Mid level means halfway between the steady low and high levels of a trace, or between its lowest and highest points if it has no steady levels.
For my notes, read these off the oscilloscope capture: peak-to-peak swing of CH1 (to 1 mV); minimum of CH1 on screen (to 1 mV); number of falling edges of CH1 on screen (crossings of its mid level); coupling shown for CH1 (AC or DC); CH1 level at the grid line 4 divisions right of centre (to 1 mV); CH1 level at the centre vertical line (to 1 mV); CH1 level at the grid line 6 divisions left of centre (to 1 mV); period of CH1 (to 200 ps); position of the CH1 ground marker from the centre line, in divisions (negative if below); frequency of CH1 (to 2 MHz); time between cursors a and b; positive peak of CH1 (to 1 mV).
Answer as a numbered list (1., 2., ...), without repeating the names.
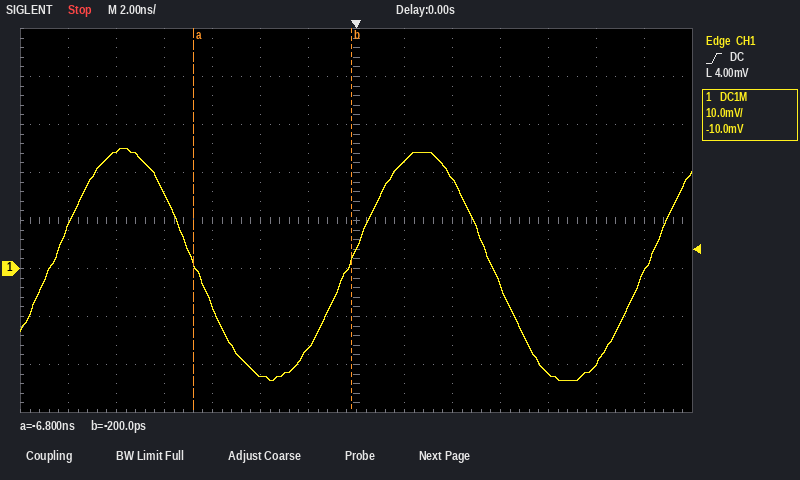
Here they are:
1. 48 mV
2. -23 mV
3. 2
4. DC
5. -22 mV
6. 4 mV
7. 9 mV
8. 12.4 ns
9. -1.0 div
10. 80 MHz
11. 6.6 ns
12. 25 mV
